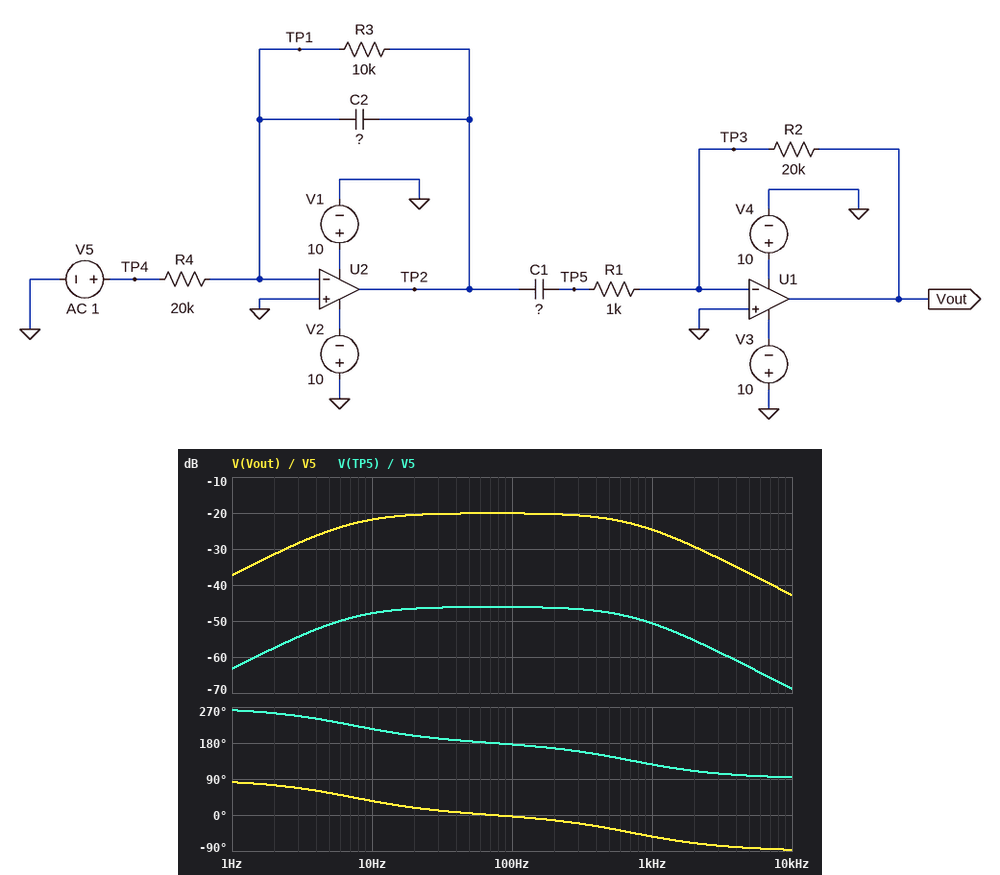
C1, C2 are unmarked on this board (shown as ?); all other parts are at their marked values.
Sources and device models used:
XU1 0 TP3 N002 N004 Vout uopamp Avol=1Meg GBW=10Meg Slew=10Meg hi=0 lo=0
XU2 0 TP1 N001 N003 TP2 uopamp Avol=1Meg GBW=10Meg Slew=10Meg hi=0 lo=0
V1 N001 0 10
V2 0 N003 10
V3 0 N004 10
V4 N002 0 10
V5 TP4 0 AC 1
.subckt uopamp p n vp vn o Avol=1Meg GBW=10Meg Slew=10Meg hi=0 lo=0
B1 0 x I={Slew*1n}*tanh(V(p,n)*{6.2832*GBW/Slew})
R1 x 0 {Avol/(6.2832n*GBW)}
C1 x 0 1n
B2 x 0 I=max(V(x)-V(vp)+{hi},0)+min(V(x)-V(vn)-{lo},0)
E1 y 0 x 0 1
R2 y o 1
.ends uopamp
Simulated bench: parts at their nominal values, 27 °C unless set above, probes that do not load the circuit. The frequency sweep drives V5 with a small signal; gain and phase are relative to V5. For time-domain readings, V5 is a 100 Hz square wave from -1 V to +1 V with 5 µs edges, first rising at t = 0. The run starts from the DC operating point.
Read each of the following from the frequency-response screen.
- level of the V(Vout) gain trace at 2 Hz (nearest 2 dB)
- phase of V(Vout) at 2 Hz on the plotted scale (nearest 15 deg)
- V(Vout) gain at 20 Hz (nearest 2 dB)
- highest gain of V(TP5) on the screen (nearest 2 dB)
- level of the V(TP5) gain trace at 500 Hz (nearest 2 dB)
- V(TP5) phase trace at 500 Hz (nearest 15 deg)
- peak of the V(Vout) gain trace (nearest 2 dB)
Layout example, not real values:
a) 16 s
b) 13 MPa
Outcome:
a) -32 dB
b) 75 deg
c) -20 dB
d) -46 dB
e) -48 dB
f) 150 deg
g) -20 dB
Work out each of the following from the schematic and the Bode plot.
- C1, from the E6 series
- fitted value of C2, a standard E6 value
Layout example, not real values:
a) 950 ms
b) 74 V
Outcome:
a) 220 nF
b) 2.2 µF
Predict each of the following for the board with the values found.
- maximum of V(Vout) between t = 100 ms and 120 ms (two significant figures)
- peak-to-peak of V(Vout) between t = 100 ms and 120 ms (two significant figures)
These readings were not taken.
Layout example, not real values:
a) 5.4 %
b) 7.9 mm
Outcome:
a) 110 mV
b) 210 mV
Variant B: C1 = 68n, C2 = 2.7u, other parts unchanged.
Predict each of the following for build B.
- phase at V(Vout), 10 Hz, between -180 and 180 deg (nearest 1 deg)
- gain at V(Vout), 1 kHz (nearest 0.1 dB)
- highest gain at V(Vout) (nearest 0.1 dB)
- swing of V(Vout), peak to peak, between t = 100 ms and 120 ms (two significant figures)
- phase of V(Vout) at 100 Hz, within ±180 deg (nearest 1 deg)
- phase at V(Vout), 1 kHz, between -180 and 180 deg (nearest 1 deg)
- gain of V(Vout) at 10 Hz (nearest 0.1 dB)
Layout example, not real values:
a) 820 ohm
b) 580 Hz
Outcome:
a) 30 deg
b) -32.7 dB
c) -32.0 dB
d) 54 mV
e) 1 deg
f) -23 deg
g) -33.3 dB
